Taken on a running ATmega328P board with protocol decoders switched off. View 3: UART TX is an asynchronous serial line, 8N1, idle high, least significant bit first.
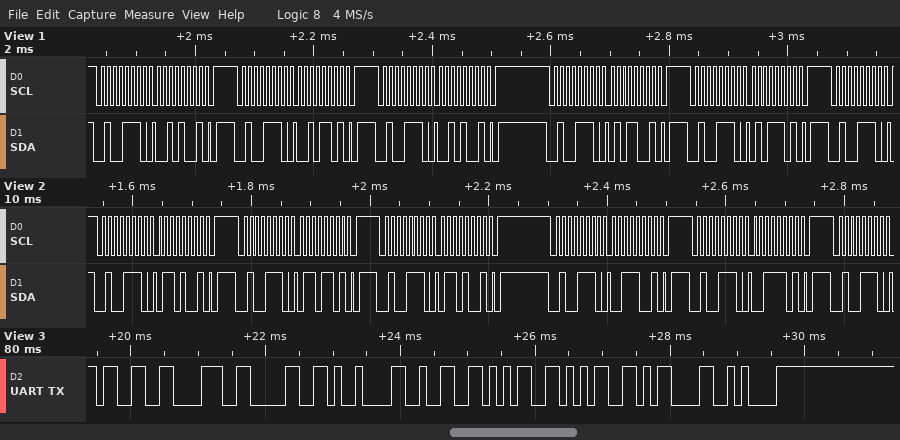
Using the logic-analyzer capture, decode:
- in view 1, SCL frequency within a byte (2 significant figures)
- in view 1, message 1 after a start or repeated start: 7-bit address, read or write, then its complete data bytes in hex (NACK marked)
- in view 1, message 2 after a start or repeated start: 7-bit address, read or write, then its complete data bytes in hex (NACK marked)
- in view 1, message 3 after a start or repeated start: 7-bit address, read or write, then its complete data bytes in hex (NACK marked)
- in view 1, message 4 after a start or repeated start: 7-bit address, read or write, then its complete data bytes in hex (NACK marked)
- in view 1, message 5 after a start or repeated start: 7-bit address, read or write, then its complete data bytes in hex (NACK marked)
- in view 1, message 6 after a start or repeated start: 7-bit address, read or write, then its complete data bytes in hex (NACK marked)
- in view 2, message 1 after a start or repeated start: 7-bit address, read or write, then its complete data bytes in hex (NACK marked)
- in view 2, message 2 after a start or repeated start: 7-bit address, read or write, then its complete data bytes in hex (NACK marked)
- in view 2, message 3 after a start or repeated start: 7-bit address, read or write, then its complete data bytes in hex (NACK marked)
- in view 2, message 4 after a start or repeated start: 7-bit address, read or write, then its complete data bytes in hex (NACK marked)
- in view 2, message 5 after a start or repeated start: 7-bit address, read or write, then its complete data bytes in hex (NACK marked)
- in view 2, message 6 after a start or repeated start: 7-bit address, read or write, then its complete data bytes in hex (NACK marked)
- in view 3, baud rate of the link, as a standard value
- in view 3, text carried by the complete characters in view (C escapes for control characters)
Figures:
100 kHz
0x27 write: 29
0x27 write: 2D
0x27 write: 29
0x27 write: 59
0x27 write: 5D
0x27 write
0x27 write: 69
0x27 write: 6D
0x27 write: 69
0x27 write: 39
0x27 write: 3D
0x27 write
9600 baud
"380\t255\r\n"
